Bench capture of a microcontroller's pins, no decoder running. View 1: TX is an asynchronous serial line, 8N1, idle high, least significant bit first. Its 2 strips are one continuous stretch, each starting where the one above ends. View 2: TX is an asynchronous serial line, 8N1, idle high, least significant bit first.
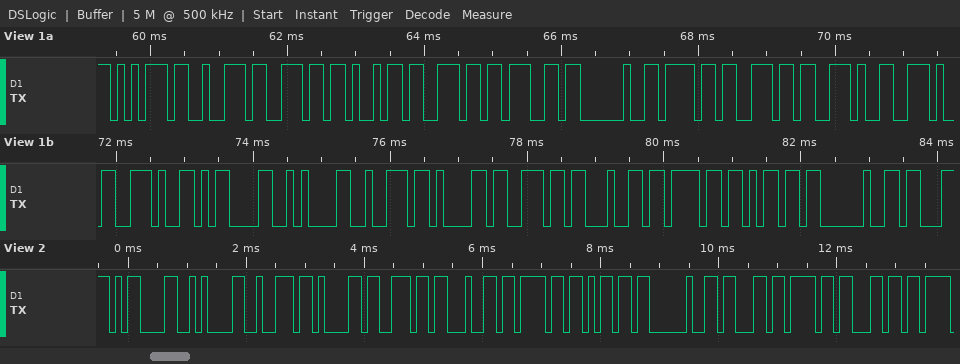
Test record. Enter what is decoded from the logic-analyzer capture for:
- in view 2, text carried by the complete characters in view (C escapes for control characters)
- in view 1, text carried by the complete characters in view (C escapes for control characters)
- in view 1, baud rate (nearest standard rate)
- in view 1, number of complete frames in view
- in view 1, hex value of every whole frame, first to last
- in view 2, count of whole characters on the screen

"\r\nrandom col"
"urning on...\r\nrandom "
9600 baud
21
75 72 6E 69 6E 67 20 6F 6E 2E 2E 2E 0D 0A 72 61 6E 64 6F 6D 20
12
